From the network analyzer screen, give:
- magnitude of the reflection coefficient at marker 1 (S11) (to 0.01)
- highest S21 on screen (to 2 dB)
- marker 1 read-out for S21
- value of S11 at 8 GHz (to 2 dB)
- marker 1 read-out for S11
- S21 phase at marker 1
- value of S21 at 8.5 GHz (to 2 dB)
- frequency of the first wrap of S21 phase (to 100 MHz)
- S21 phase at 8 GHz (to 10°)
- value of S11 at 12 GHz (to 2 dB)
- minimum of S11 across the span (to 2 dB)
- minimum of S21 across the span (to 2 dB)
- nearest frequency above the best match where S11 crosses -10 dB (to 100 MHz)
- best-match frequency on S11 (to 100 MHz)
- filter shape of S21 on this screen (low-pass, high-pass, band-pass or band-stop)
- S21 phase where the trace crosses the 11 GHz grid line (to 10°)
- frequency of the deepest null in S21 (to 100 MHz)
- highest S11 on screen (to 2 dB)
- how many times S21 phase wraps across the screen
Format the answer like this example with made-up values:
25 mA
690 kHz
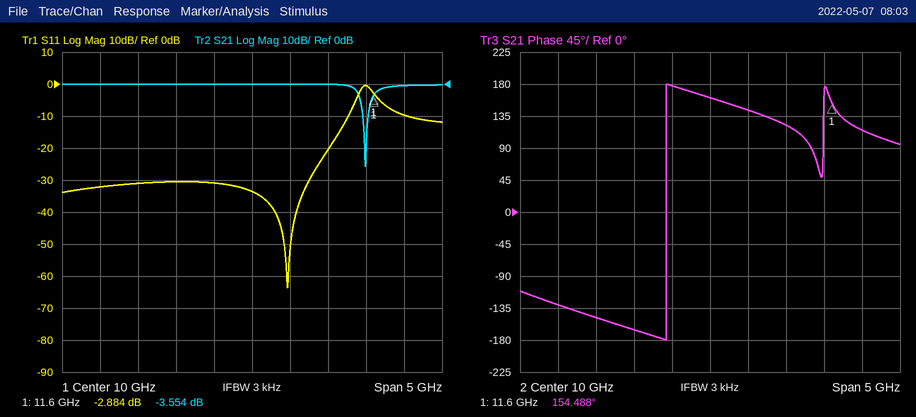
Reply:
0.72
0 dB
-3.554 dB
-32 dB
-2.884 dB
154.488°
0 dB
9.4 GHz
-130°
-10 dB
-64 dB
-26 dB
11.3 GHz
10.5 GHz
band-stop
120°
11.5 GHz
0 dB
1
